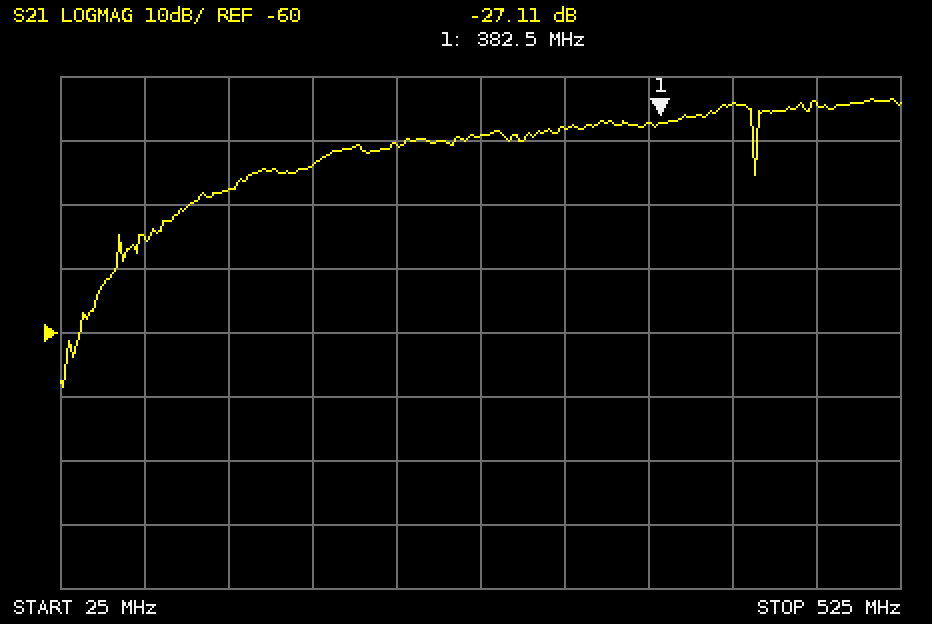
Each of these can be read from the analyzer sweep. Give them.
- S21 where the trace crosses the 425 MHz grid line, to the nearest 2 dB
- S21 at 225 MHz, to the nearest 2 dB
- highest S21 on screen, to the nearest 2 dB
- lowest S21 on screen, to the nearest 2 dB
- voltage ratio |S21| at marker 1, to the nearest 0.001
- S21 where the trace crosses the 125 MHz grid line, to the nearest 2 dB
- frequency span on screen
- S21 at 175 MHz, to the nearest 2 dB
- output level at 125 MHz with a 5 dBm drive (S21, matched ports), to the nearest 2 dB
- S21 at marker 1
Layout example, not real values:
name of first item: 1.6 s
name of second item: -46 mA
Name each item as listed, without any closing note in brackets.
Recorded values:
S21 where the trace crosses the 425 MHz grid line, to the nearest 2 dB: -24 dB
S21 at 225 MHz, to the nearest 2 dB: -30 dB
highest S21 on screen, to the nearest 2 dB: -24 dB
lowest S21 on screen, to the nearest 2 dB: -68 dB
voltage ratio |S21| at marker 1, to the nearest 0.001: 0.044
S21 where the trace crosses the 125 MHz grid line, to the nearest 2 dB: -38 dB
frequency span on screen: 500 MHz
S21 at 175 MHz, to the nearest 2 dB: -34 dB
output level at 125 MHz with a 5 dBm drive (S21, matched ports), to the nearest 2 dB: -32 dBm
S21 at marker 1: -27.11 dB
